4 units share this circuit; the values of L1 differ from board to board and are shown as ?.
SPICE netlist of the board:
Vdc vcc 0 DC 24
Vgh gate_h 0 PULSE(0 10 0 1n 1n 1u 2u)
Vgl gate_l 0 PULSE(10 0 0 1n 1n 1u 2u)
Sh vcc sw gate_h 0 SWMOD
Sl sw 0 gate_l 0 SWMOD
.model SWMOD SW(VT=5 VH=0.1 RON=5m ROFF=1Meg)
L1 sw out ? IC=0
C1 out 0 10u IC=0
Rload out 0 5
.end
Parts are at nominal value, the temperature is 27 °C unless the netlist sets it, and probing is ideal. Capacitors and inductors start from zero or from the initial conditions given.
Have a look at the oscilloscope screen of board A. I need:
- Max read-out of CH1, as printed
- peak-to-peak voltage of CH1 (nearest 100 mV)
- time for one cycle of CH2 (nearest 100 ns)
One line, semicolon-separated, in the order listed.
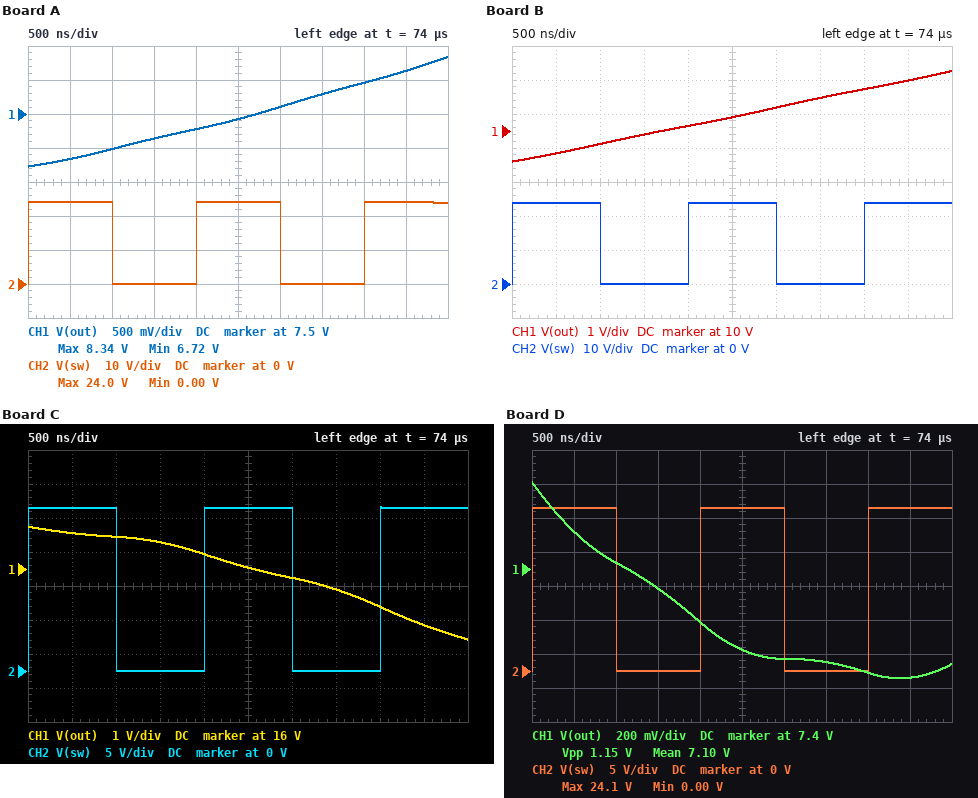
8.34 V; 1.6 V; 2.0 µs
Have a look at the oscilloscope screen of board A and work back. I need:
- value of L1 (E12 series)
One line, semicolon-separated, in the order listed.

12 µH
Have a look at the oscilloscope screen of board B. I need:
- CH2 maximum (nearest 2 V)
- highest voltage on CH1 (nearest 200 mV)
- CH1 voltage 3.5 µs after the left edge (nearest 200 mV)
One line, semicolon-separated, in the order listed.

24 V; 11.8 V; 11.0 V
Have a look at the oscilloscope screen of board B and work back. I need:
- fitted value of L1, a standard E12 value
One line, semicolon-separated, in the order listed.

10 µH
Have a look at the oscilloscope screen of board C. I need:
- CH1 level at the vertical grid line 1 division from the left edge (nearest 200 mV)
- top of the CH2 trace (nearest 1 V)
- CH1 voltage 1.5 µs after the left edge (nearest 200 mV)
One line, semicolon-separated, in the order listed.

17.0 V; 24 V; 16.8 V
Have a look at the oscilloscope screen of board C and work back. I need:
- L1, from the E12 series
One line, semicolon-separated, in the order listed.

2.2 µH
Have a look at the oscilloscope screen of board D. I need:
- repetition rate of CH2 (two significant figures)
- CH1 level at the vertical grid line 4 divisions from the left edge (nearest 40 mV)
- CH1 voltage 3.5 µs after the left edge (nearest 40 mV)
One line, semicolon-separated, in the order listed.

500 kHz; 7.08 V; 6.84 V
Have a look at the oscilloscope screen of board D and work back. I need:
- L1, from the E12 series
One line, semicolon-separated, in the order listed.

3.9 µH
